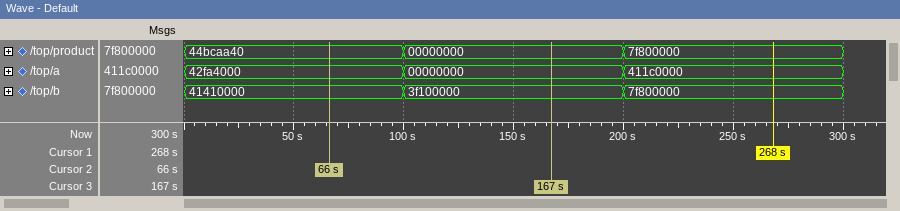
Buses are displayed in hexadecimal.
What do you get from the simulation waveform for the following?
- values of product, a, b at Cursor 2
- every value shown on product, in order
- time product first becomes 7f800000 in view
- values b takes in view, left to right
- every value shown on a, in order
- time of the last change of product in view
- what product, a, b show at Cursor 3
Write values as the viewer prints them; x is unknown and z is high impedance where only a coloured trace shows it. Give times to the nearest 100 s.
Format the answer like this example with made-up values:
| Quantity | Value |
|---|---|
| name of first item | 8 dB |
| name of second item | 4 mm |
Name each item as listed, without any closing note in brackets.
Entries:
| Quantity | Value |
|---|---|
| values of product, a, b at Cursor 2 | product=44bcaa40, a=42fa4000, b=41410000 |
| every value shown on product, in order | 44bcaa40, 00000000, 7f800000 |
| time product first becomes 7f800000 in view | 200 s |
| values b takes in view, left to right | 41410000, 3f100000, 7f800000 |
| every value shown on a, in order | 42fa4000, 00000000, 411c0000 |
| time of the last change of product in view | 200 s |
| what product, a, b show at Cursor 3 | product=00000000, a=00000000, b=3f100000 |
